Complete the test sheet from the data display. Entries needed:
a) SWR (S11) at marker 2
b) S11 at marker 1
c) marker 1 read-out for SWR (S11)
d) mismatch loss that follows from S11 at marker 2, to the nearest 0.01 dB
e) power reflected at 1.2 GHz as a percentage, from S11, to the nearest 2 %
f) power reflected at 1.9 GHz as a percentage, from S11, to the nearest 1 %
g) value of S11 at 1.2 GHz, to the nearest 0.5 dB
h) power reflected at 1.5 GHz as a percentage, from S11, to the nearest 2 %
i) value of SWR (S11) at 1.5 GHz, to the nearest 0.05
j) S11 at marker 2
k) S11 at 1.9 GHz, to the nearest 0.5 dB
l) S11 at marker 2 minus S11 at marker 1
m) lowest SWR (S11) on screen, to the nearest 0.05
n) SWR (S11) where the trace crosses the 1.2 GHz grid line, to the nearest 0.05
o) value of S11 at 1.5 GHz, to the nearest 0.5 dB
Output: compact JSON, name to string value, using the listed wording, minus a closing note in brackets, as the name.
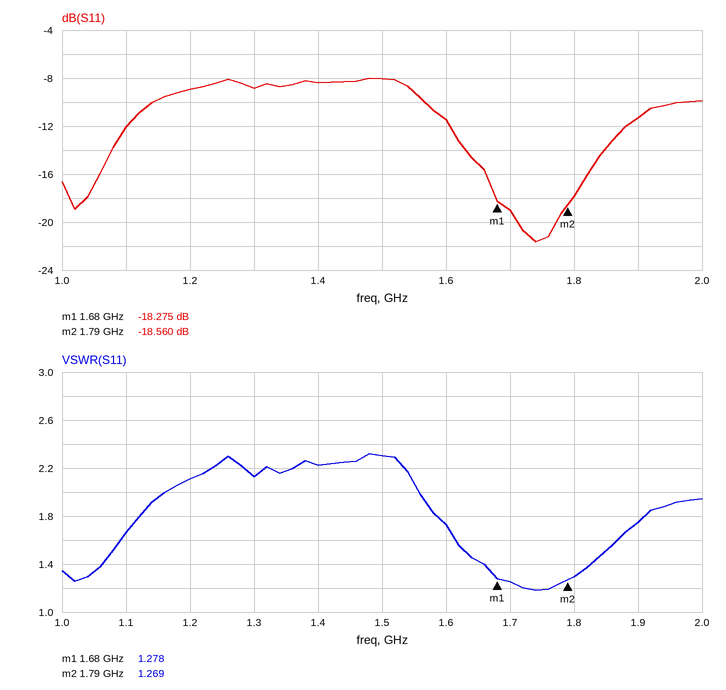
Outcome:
{"SWR (S11) at marker 2": "1.269", "S11 at marker 1": "-18.275 dB", "marker 1 read-out for SWR": "1.278", "mismatch loss that follows from S11 at marker 2, to the nearest 0.01 dB": "0.06 dB", "power reflected at 1.2 GHz as a percentage, from S11, to the nearest 2 %": "12 %", "power reflected at 1.9 GHz as a percentage, from S11, to the nearest 1 %": "7 %", "value of S11 at 1.2 GHz, to the nearest 0.5 dB": "-9.0 dB", "power reflected at 1.5 GHz as a percentage, from S11, to the nearest 2 %": "16 %", "value of SWR (S11) at 1.5 GHz, to the nearest 0.05": "2.30", "S11 at marker 2": "-18.560 dB", "S11 at 1.9 GHz, to the nearest 0.5 dB": "-11.5 dB", "S11 at marker 2 minus S11 at marker 1": "-0.285 dB", "lowest SWR (S11) on screen, to the nearest 0.05": "1.20", "SWR (S11) where the trace crosses the 1.2 GHz grid line, to the nearest 0.05": "2.10", "value of S11 at 1.5 GHz, to the nearest 0.5 dB": "-8.0 dB"}
